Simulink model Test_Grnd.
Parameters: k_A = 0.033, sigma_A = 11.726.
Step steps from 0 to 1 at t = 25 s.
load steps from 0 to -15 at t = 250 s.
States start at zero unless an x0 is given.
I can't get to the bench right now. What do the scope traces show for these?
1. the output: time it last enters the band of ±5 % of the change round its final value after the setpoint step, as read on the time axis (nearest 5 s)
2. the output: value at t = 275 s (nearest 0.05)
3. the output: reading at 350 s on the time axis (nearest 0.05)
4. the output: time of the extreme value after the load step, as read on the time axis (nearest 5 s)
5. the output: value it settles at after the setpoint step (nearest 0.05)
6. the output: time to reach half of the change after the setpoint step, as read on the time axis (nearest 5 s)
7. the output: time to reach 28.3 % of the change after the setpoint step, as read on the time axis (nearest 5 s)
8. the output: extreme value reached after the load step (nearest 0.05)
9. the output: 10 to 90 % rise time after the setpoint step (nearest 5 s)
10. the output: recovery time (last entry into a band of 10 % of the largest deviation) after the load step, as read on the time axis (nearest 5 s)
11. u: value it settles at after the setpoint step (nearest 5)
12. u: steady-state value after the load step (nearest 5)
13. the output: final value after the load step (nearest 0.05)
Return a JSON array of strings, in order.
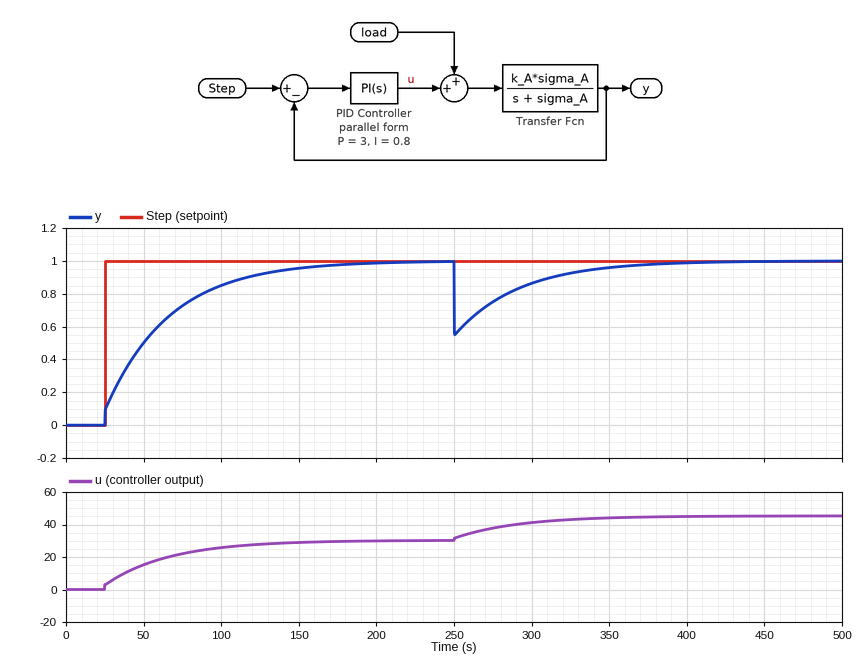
["145 s", "0.75", "0.95", "250 s", "1.00", "50 s", "35 s", "0.55", "90 s", "345 s", "30", "45", "1.00"]
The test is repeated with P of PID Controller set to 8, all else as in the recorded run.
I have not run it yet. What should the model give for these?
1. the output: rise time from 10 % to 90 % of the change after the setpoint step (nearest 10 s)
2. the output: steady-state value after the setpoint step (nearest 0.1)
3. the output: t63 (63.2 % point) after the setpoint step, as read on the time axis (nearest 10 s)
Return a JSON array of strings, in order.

["100 s", "1.0", "60 s"]
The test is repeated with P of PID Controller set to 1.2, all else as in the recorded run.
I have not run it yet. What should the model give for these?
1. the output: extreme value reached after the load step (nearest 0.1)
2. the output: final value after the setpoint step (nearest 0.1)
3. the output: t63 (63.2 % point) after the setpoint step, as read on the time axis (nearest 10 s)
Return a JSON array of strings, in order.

["0.5", "1.0", "60 s"]
